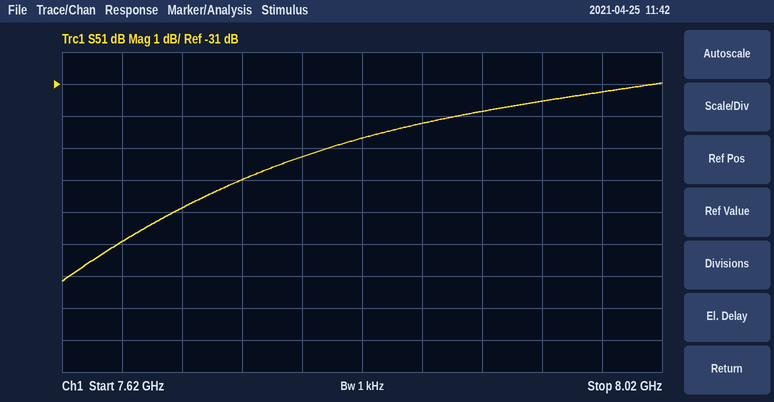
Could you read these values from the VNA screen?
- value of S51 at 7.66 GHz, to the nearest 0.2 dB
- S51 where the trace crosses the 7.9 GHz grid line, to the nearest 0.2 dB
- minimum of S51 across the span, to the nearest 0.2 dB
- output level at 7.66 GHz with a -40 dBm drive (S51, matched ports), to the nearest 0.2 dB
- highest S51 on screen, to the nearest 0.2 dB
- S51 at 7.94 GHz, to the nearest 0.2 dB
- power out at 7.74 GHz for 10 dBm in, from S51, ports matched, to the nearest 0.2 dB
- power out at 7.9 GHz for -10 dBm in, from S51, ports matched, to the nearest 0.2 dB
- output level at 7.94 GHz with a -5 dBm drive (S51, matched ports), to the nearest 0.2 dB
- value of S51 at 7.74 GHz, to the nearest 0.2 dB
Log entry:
-36.0 dB
-31.8 dB
-37.2 dB
-76.0 dBm
-31.0 dB
-31.6 dB
-24.0 dBm
-41.8 dBm
-36.6 dBm
-34.0 dB
